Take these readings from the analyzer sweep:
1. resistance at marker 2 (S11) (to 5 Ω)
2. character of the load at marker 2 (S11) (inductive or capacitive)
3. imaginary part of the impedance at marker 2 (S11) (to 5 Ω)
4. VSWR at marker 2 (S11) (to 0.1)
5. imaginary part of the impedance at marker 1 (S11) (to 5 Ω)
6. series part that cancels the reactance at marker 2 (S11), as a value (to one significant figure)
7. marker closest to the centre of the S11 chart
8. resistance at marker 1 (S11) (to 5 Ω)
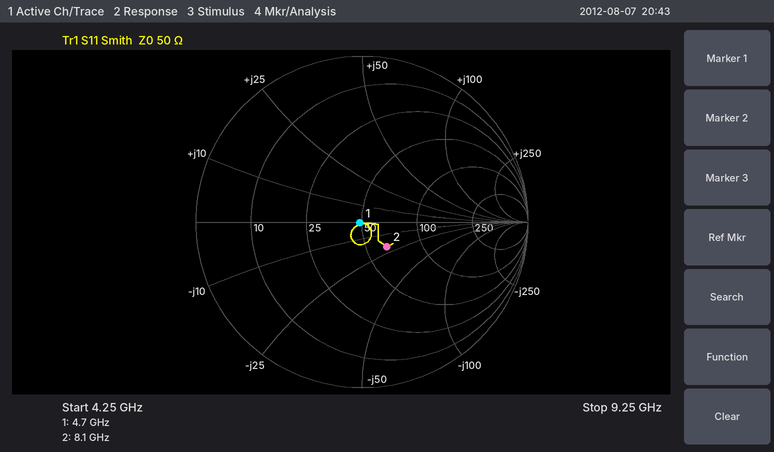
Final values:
65 Ω
capacitive
-20 Ω
1.5
0 Ω
400 pH
marker 1
50 Ω
